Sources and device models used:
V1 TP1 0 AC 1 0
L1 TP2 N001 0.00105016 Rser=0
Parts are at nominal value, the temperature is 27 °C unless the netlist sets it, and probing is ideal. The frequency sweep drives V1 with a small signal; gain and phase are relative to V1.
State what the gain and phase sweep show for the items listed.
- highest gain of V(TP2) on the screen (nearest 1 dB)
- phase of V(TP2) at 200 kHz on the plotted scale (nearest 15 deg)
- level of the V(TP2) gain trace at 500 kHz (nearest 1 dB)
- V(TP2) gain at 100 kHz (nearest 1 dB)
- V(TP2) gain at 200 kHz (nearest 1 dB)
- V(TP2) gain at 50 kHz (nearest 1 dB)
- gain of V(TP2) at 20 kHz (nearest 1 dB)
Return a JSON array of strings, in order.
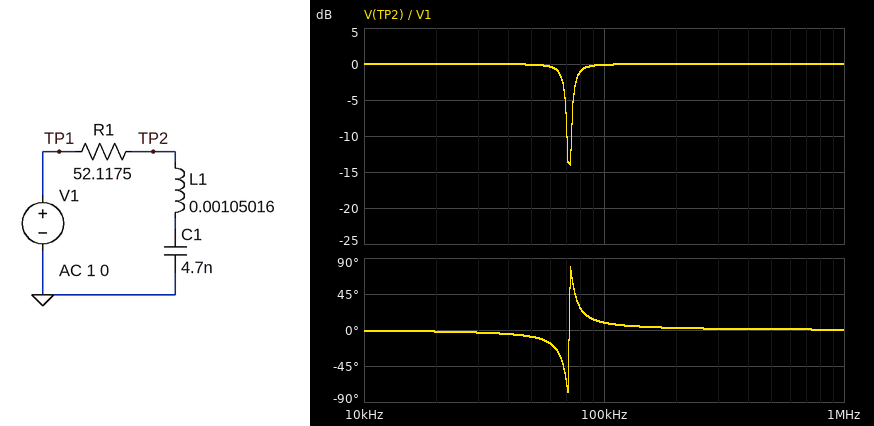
["0 dB", "0 deg", "0 dB", "0 dB", "0 dB", "0 dB", "0 dB"]
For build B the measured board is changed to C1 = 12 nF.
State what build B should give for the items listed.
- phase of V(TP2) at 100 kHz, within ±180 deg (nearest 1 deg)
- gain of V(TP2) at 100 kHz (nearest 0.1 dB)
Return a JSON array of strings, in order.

["6 deg", "0 dB"]
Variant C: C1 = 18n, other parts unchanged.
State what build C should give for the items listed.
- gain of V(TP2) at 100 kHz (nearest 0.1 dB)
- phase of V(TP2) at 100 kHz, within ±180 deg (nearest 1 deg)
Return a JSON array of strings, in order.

["0 dB", "5 deg"]
